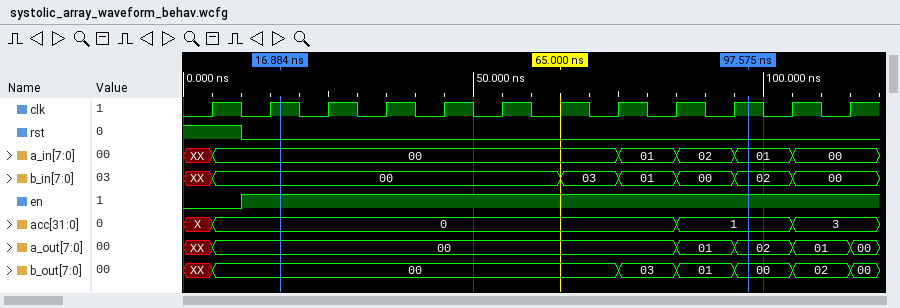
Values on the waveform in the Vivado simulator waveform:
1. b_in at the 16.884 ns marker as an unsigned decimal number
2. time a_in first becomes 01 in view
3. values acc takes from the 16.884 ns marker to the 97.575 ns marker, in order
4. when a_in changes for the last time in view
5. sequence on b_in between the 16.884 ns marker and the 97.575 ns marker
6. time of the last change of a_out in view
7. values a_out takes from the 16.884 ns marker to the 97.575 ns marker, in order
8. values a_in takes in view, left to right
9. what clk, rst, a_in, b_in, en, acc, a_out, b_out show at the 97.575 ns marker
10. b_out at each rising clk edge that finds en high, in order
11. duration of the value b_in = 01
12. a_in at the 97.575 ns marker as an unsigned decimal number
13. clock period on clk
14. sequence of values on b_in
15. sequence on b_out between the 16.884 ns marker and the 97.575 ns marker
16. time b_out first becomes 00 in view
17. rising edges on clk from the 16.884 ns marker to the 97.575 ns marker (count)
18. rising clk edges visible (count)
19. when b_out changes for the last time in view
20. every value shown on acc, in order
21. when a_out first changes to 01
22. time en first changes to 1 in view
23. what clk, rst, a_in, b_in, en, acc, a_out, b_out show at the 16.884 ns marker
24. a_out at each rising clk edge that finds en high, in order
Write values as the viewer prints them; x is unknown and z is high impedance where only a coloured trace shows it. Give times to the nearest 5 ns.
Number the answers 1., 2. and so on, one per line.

1. 0
2. 75 ns
3. 0, 1
4. 105 ns
5. 00, 03, 01, 00, 02
6. 115 ns
7. 00, 01, 02
8. XX, 00, 01, 02, 01, 00
9. clk=1, rst=0, a_in=01, b_in=02, en=1, acc=1, a_out=02, b_out=00
10. 00, 00, 00, 00, 00, 00, 00, 03, 01, 00, 02
11. 10 ns
12. 1
13. 10 ns
14. XX, 00, 03, 01, 00, 02, 00
15. 00, 03, 01, 00
16. 5 ns
17. 8
18. 12
19. 115 ns
20. X, 0, 1, 3
21. 85 ns
22. 10 ns
23. clk=1, rst=0, a_in=00, b_in=00, en=1, acc=0, a_out=00, b_out=00
24. 00, 00, 00, 00, 00, 00, 00, 00, 01, 02, 01
